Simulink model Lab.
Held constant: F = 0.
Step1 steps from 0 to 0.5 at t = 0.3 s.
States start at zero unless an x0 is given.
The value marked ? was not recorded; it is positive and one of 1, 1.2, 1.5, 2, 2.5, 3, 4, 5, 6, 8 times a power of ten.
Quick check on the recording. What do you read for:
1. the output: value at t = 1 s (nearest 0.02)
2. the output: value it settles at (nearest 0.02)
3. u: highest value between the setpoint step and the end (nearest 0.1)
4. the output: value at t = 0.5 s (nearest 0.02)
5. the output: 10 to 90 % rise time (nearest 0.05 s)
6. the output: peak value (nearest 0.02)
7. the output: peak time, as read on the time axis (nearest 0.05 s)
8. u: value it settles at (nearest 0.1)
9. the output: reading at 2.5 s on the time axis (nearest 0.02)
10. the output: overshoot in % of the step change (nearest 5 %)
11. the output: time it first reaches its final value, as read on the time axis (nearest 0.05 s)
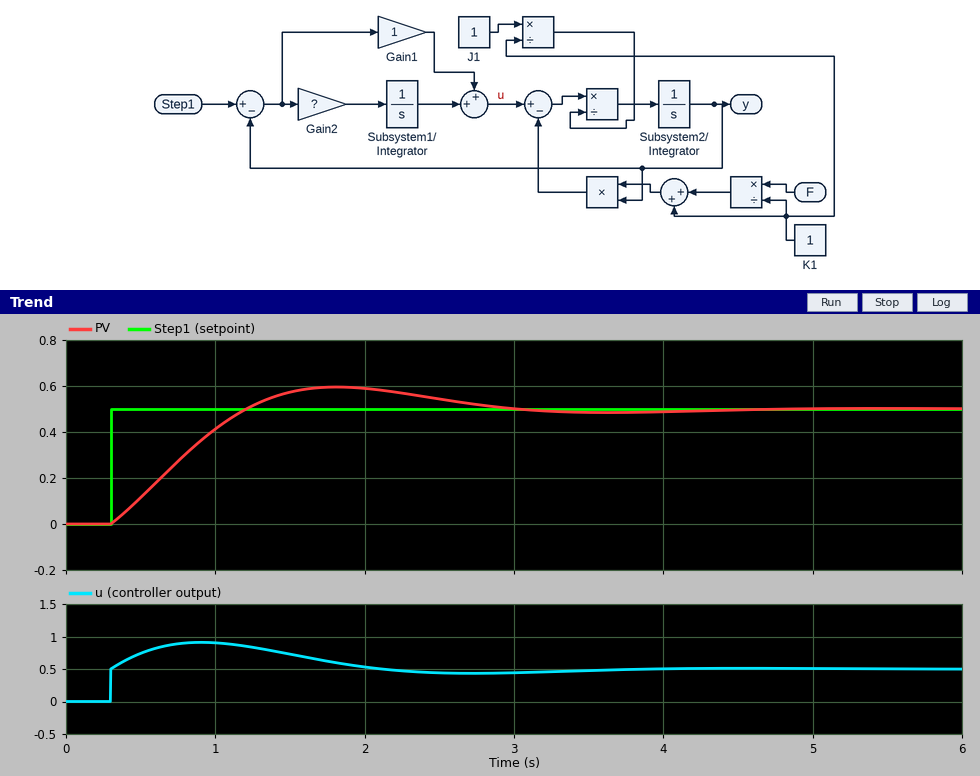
0.42
0.50
0.9
0.12
0.70 s
0.60
1.80 s
0.5
0.54
20 %
1.20 s
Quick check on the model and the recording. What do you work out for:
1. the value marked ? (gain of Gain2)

4
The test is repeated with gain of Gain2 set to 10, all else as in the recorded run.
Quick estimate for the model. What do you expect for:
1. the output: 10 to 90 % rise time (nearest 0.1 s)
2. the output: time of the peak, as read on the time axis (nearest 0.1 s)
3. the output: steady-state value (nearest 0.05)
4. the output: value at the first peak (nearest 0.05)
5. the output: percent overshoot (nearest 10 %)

0.4 s
1.2 s
0.50
0.70
40 %
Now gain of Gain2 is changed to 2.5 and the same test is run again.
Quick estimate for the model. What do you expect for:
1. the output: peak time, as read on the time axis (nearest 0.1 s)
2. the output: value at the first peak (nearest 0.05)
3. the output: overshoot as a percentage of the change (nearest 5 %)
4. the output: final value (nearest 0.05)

2.3 s
0.55
10 %
0.50
